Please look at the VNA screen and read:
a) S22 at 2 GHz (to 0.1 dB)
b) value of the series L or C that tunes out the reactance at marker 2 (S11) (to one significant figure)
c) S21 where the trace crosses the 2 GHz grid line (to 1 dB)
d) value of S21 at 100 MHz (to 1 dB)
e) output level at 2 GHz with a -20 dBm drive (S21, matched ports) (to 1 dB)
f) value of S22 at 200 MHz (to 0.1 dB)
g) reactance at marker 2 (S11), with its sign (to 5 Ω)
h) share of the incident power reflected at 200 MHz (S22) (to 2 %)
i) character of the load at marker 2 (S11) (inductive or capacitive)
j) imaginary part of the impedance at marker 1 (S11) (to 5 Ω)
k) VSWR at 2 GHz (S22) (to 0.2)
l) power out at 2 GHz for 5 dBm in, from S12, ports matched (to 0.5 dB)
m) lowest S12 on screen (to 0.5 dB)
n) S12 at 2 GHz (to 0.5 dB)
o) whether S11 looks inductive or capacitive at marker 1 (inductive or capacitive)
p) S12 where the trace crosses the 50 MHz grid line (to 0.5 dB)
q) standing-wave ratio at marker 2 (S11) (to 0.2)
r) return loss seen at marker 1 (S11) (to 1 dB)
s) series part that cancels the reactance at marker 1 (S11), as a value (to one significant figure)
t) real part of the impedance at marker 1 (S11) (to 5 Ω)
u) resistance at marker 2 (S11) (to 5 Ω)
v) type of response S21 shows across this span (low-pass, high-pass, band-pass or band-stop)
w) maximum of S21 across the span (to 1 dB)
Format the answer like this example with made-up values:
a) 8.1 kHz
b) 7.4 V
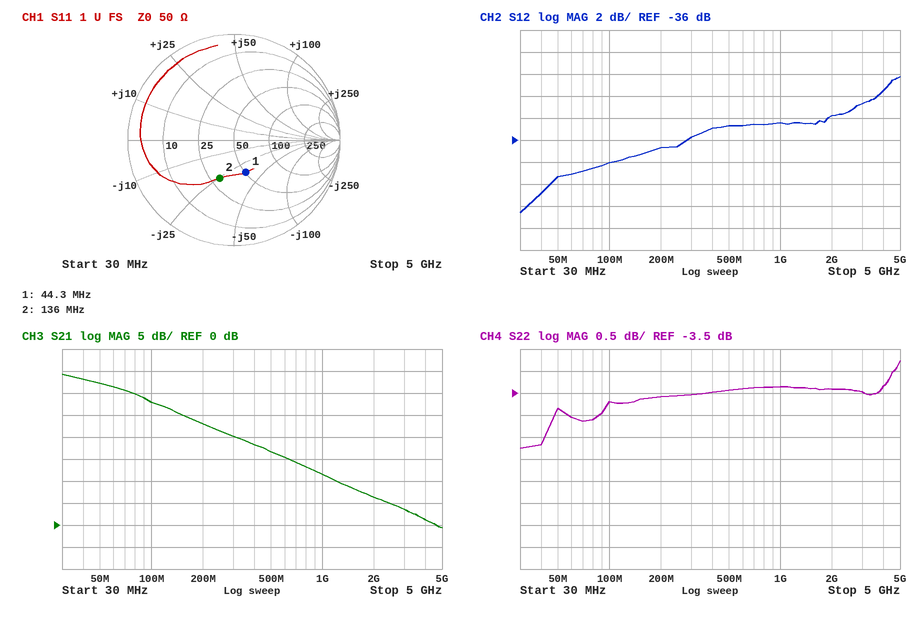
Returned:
a) -3.4 dB
b) 30 nH
c) 6 dB
d) 28 dB
e) -14 dBm
f) -3.6 dB
g) -25 Ω
h) 44 %
i) capacitive
j) -35 Ω
k) 5.2
l) -29.0 dBm
m) -42.5 dB
n) -34.0 dB
o) capacitive
p) -39.5 dB
q) 2.2
r) 10 dB
s) 100 nH
t) 50 Ω
u) 30 Ω
v) low-pass
w) 34 dB
